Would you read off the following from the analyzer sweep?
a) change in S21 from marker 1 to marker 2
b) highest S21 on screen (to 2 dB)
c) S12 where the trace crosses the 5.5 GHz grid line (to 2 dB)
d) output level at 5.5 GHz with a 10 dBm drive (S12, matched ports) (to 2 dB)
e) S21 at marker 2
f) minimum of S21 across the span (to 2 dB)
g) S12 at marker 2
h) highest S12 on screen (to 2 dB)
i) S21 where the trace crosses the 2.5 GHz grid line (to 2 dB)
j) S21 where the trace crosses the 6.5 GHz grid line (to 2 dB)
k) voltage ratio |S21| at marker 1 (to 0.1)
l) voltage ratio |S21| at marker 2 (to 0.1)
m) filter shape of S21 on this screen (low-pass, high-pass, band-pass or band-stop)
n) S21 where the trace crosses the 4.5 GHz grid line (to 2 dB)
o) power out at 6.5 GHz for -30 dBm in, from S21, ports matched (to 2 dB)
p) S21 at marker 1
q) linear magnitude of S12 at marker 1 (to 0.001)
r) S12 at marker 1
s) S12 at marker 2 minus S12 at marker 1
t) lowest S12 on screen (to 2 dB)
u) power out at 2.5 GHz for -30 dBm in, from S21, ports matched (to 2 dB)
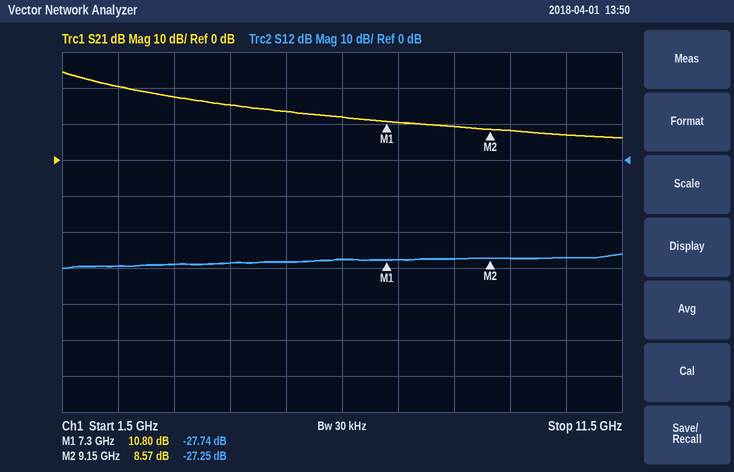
-2.23 dB
24 dB
-28 dB
-18 dBm
8.57 dB
6 dB
-27.25 dB
-26 dB
20 dB
12 dB
3.5
2.7
low-pass
16 dB
-18 dBm
10.80 dB
0.041
-27.74 dB
0.49 dB
-30 dB
-10 dBm
